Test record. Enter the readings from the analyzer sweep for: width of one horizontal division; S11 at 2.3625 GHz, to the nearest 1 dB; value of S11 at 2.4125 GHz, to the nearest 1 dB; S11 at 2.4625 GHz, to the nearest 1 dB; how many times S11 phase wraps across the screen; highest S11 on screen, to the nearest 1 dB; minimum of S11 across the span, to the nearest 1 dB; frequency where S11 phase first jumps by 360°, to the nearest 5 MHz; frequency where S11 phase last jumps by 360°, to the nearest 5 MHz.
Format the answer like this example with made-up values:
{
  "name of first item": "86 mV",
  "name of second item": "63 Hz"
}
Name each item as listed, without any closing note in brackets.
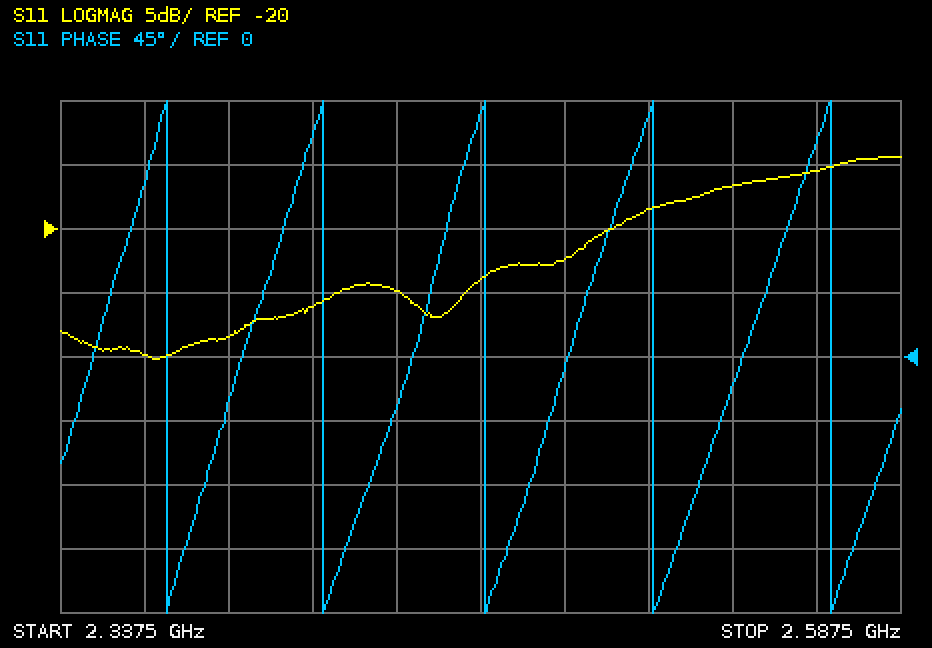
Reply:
{
  "width of one horizontal division": "25 MHz",
  "S11 at 2.3625 GHz, to the nearest 1 dB": "-30 dB",
  "value of S11 at 2.4125 GHz, to the nearest 1 dB": "-26 dB",
  "S11 at 2.4625 GHz, to the nearest 1 dB": "-24 dB",
  "how many times S11 phase wraps across the screen": "5",
  "highest S11 on screen, to the nearest 1 dB": "-14 dB",
  "minimum of S11 across the span, to the nearest 1 dB": "-30 dB",
  "frequency where S11 phase first jumps by 360°, to the nearest 5 MHz": "2.370 GHz",
  "frequency where S11 phase last jumps by 360°, to the nearest 5 MHz": "2.565 GHz"
}
